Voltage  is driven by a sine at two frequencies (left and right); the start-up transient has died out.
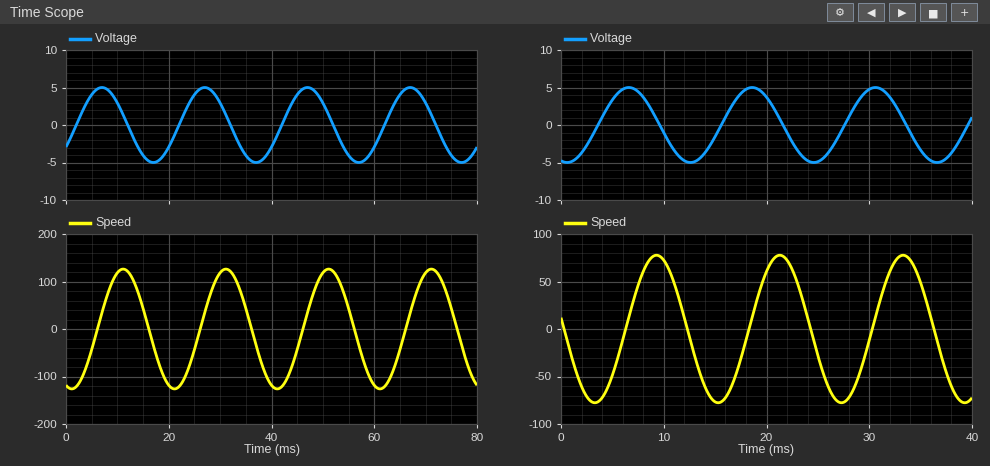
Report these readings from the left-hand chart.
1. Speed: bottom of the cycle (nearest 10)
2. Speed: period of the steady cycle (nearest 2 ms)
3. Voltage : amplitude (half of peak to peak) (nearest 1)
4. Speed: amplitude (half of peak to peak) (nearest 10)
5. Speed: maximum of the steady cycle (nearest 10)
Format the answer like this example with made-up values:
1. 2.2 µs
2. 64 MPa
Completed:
1. -130
2. 20 ms
3. 5
4. 130
5. 130
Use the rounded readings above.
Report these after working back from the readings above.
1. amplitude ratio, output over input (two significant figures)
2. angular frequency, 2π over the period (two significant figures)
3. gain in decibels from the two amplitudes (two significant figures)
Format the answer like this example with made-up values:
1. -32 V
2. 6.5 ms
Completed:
1. 26
2. 0.31 rad/ms
3. 28 dB
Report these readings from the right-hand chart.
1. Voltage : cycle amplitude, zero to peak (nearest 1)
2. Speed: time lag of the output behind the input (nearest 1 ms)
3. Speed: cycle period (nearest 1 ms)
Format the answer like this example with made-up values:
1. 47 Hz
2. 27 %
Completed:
1. 5
2. 3 ms
3. 12 ms
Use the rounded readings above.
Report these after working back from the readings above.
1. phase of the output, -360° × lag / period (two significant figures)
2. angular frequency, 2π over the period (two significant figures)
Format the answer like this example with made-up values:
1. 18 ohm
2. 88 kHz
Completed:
1. -90°
2. 0.52 rad/ms
